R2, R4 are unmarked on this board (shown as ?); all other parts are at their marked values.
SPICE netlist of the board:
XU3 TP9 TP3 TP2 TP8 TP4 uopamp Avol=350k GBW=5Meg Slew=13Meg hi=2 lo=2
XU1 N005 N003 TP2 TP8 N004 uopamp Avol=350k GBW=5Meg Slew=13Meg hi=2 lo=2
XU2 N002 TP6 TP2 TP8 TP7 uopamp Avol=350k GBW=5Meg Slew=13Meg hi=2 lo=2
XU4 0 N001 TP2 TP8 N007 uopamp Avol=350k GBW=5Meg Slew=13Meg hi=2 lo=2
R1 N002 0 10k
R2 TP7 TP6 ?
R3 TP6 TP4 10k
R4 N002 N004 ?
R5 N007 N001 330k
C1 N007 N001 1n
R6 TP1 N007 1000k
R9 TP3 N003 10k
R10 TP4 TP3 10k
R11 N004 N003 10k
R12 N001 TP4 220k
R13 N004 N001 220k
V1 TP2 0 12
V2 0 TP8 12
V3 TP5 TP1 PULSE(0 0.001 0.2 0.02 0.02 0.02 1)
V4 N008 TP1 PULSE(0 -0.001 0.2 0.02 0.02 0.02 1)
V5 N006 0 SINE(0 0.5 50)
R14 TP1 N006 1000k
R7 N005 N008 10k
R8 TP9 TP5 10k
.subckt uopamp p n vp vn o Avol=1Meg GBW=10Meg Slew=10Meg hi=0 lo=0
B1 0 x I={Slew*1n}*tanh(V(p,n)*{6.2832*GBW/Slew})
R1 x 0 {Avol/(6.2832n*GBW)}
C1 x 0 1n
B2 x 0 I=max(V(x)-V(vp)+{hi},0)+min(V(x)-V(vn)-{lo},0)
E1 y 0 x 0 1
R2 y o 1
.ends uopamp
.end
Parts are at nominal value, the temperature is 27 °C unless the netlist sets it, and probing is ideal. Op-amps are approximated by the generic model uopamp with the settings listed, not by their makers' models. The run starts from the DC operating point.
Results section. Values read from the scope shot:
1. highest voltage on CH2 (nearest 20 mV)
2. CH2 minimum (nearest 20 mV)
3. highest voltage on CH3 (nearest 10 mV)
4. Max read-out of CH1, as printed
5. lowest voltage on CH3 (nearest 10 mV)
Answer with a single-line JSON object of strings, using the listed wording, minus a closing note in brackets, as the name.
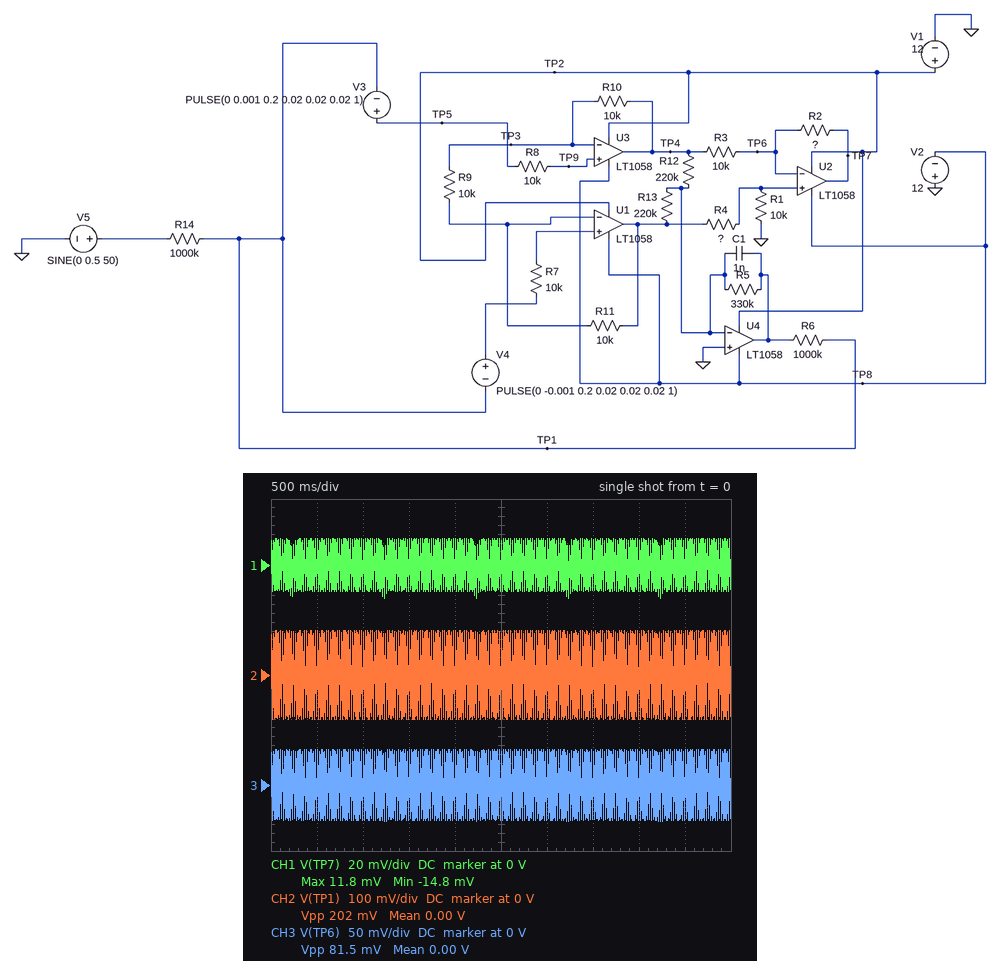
{"highest voltage on CH2": "100 mV", "CH2 minimum": "-100 mV", "highest voltage on CH3": "40 mV", "Max read-out of CH1, as printed": "11.8 mV", "lowest voltage on CH3": "-40 mV"}
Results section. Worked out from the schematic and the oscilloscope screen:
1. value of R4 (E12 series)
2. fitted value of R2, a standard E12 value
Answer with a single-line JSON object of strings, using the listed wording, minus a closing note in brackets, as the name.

{"value of R4": "15 kΩ", "fitted value of R2, a standard E12 value": "4.7 kΩ"}
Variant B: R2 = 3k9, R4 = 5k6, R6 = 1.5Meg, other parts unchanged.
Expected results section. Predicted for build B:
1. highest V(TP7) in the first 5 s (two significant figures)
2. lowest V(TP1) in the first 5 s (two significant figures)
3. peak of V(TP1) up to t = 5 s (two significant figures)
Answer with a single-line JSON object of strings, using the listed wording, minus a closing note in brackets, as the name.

{"highest V(TP7) in the first 5 s": "69 mV", "lowest V(TP1) in the first 5 s": "-140 mV", "peak of V(TP1) up to t = 5 s": "140 mV"}
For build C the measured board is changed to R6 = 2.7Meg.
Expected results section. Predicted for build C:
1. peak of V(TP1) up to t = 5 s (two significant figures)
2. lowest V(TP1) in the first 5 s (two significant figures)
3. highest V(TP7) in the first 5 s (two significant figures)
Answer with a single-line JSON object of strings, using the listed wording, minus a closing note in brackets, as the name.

{"peak of V(TP1) up to t = 5 s": "200 mV", "lowest V(TP1) in the first 5 s": "-200 mV", "highest V(TP7) in the first 5 s": "24 mV"}
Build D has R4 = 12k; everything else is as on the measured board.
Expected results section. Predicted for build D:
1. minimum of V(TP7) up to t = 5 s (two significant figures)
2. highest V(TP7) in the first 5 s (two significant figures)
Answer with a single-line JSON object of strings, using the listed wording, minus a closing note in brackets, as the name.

{"minimum of V(TP7) up to t = 5 s": "-23 mV", "highest V(TP7) in the first 5 s": "20 mV"}
